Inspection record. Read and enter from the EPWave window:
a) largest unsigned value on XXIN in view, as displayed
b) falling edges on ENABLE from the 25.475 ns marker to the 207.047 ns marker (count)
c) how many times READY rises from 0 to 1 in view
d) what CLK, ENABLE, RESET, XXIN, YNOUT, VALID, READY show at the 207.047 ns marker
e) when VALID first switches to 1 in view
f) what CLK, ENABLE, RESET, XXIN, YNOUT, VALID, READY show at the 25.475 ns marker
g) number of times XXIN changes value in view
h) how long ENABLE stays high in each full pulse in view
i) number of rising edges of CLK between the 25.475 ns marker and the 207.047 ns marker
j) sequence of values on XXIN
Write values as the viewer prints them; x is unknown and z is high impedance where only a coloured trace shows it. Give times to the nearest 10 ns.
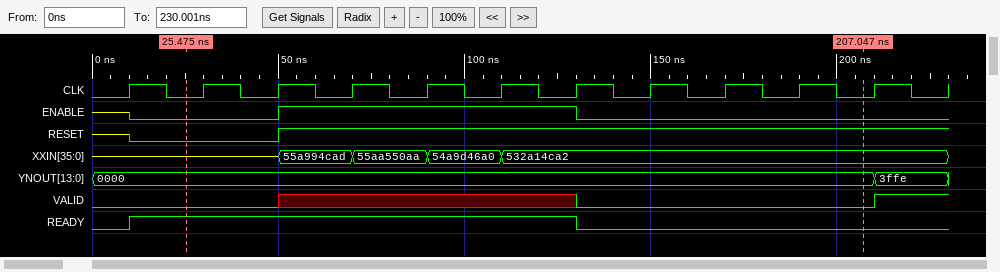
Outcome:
55aa550aa
1
1
CLK=0, ENABLE=0, RESET=1, XXIN=532a14ca2, YNOUT=0000, VALID=0, READY=0
210 ns
CLK=0, ENABLE=0, RESET=0, XXIN=z, YNOUT=0000, VALID=0, READY=1
4
80 ns
9
z, 55a994cad, 55aa550aa, 54a9d46a0, 532a14ca2
